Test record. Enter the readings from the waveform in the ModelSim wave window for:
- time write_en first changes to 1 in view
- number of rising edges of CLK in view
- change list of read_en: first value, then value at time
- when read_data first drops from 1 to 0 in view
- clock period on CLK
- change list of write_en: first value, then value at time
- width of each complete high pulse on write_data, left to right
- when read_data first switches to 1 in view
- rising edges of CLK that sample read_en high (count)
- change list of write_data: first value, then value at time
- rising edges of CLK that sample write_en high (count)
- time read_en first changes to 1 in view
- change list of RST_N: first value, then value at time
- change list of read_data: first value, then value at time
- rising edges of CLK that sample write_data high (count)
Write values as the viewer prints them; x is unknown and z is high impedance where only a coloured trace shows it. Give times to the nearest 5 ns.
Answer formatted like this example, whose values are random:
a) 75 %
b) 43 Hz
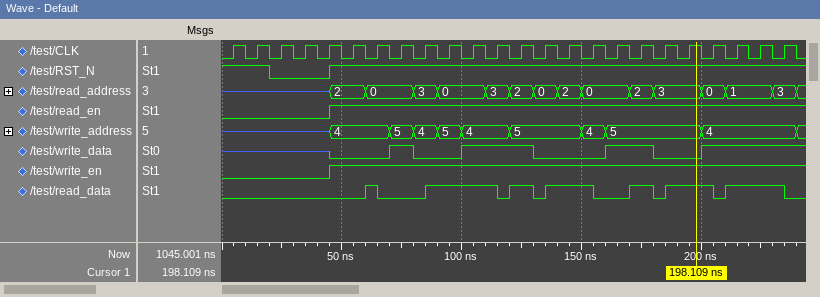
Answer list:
a) 45 ns
b) 24
c) 0, 1 at 45 ns
d) 65 ns
e) 10 ns
f) 0, 1 at 45 ns
g) 10 ns, 30 ns, 20 ns
h) 60 ns
i) 19
j) z, 0 at 45 ns, 1 at 70 ns, 0 at 80 ns, 1 at 100 ns, 0 at 130 ns, 1 at 160 ns, 0 at 180 ns, 1 at 200 ns
k) 19
l) 45 ns
m) 1, 0 at 20 ns, 1 at 45 ns
n) 0, 1 at 60 ns, 0 at 65 ns, 1 at 85 ns, 0 at 115 ns, 1 at 120 ns, 0 at 130 ns, 1 at 135 ns, 0 at 155 ns, 1 at 170 ns, 0 at 180 ns, 1 at 185 ns, 0 at 205 ns, 1 at 210 ns, 0 at 235 ns
o) 10
